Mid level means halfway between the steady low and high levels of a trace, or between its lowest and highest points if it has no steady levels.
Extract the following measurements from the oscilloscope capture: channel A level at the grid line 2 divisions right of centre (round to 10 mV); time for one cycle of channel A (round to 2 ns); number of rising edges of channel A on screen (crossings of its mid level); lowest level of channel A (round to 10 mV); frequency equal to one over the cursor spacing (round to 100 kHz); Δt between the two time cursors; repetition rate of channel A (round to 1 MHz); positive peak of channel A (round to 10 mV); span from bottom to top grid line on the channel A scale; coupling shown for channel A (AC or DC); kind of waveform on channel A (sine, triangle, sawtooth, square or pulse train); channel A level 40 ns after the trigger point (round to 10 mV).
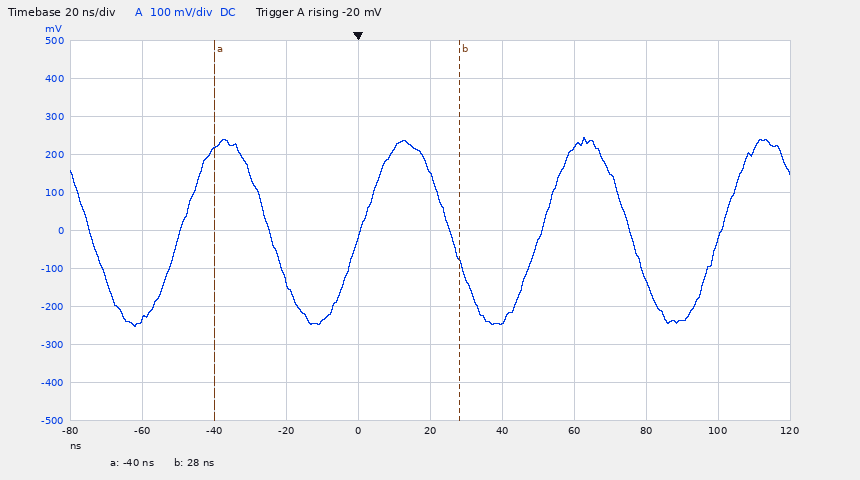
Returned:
220 mV
50 ns
4
-250 mV
14.7 MHz
68 ns
20 MHz
240 mV
1 V
DC
sine
-240 mV
